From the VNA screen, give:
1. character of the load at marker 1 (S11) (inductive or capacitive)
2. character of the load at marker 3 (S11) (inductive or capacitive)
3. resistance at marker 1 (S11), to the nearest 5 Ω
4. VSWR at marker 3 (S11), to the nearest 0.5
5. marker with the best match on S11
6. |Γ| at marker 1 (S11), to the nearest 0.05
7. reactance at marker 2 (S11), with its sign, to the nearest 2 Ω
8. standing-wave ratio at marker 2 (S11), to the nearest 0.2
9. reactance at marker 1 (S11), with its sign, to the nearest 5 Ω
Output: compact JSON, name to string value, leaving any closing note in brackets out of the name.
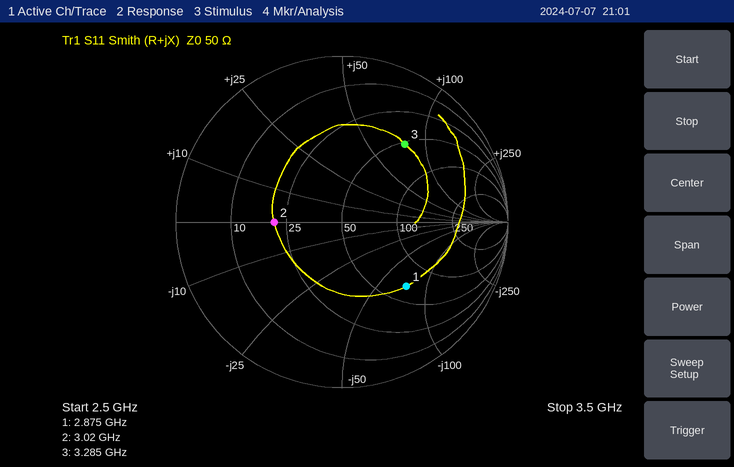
{"character of the load at marker 1 (S11)": "capacitive", "character of the load at marker 3 (S11)": "inductive", "resistance at marker 1 (S11), to the nearest 5 Ω": "65 Ω", "VSWR at marker 3 (S11), to the nearest 0.5": "4.0", "marker with the best match on S11": "marker 2", "|Γ| at marker 1 (S11), to the nearest 0.05": "0.55", "reactance at marker 2 (S11), with its sign, to the nearest 2 Ω": "0 Ω", "standing-wave ratio at marker 2 (S11), to the nearest 0.2": "2.4", "reactance at marker 1 (S11), with its sign, to the nearest 5 Ω": "-75 Ω"}
